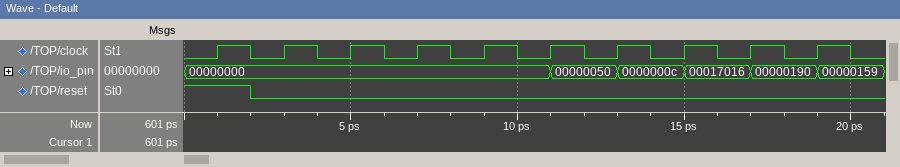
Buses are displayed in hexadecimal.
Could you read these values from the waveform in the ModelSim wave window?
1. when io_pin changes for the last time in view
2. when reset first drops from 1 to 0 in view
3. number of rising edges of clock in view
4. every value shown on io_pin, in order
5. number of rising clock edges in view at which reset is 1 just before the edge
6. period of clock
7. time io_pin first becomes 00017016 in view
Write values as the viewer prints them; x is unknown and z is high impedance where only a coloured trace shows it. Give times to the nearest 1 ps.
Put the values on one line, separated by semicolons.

19 ps; 2 ps; 10; 00000000, 00000050, 0000000c, 00017016, 00000190, 00000159; 1; 2 ps; 15 ps
